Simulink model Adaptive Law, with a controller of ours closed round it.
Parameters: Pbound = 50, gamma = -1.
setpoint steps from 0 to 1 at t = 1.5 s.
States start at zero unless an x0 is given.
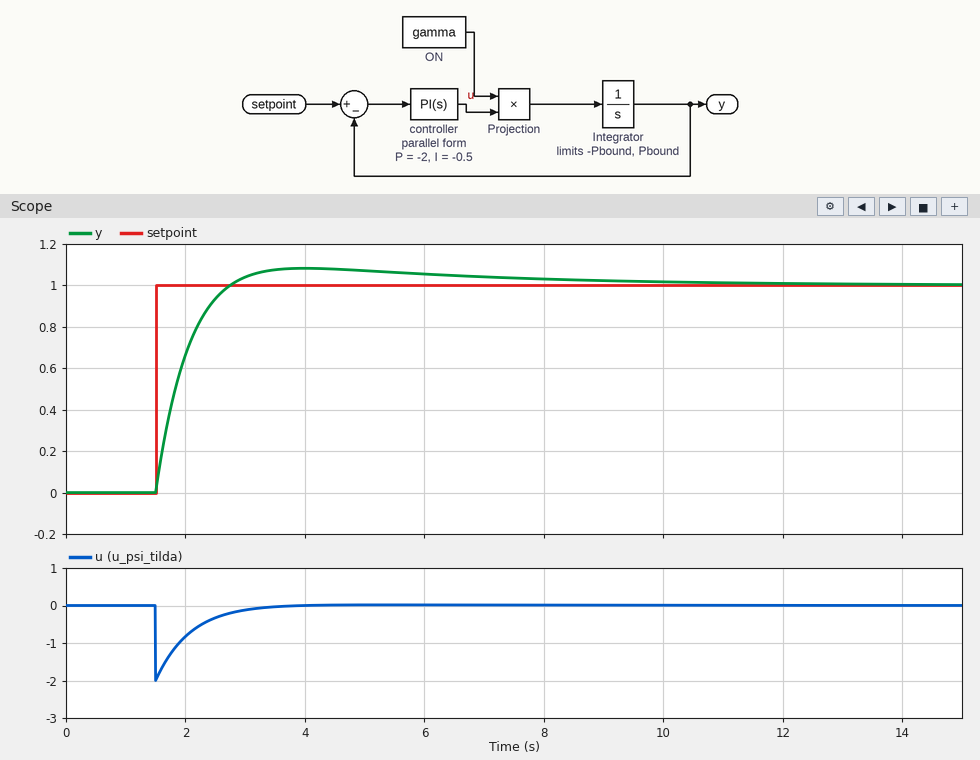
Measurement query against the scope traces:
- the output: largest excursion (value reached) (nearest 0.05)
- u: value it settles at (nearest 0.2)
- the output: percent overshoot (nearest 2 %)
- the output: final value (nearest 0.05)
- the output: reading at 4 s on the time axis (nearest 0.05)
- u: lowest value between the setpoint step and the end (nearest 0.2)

1.10
0.0
8 %
1.00
1.10
-2.0
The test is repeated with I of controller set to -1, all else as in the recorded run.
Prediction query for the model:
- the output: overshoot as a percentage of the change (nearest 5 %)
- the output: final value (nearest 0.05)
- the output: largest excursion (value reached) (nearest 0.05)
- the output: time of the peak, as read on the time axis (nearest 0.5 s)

15 %
1.00
1.15
3.5 s
